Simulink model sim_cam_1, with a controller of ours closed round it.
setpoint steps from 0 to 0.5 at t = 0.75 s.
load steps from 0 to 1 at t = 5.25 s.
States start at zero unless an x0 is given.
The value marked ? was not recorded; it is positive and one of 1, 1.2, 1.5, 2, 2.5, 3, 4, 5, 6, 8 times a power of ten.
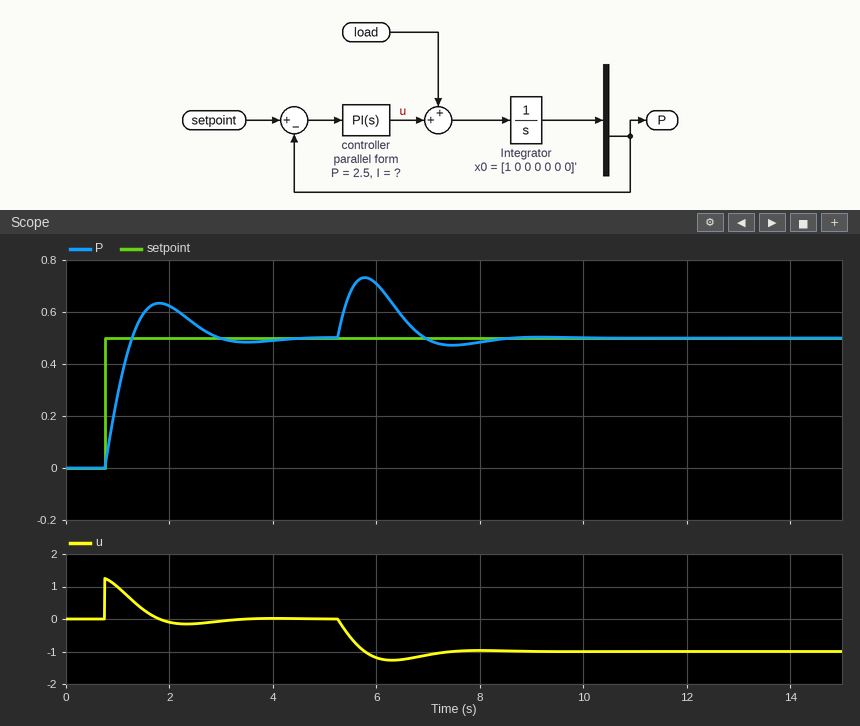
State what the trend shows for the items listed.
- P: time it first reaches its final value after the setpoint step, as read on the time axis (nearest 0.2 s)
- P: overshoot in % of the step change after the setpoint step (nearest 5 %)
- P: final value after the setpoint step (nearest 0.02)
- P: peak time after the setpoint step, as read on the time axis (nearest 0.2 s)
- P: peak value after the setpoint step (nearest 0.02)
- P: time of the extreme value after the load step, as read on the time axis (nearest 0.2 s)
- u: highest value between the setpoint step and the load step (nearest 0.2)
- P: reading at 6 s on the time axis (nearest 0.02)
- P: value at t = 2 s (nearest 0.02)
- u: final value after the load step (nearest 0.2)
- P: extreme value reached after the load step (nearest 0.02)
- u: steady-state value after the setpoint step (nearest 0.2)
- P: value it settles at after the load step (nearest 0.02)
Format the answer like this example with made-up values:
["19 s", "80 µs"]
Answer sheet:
["1.2 s", "25 %", "0.50", "1.8 s", "0.64", "5.8 s", "1.2", "0.70", "0.62", "-1.0", "0.74", "0.0", "0.50"]
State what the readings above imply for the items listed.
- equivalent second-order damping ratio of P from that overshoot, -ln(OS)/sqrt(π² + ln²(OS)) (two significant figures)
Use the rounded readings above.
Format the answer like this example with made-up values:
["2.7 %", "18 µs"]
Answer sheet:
["0.40"]
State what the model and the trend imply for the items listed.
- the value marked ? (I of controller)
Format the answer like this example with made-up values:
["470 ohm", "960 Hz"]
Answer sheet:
["5"]
